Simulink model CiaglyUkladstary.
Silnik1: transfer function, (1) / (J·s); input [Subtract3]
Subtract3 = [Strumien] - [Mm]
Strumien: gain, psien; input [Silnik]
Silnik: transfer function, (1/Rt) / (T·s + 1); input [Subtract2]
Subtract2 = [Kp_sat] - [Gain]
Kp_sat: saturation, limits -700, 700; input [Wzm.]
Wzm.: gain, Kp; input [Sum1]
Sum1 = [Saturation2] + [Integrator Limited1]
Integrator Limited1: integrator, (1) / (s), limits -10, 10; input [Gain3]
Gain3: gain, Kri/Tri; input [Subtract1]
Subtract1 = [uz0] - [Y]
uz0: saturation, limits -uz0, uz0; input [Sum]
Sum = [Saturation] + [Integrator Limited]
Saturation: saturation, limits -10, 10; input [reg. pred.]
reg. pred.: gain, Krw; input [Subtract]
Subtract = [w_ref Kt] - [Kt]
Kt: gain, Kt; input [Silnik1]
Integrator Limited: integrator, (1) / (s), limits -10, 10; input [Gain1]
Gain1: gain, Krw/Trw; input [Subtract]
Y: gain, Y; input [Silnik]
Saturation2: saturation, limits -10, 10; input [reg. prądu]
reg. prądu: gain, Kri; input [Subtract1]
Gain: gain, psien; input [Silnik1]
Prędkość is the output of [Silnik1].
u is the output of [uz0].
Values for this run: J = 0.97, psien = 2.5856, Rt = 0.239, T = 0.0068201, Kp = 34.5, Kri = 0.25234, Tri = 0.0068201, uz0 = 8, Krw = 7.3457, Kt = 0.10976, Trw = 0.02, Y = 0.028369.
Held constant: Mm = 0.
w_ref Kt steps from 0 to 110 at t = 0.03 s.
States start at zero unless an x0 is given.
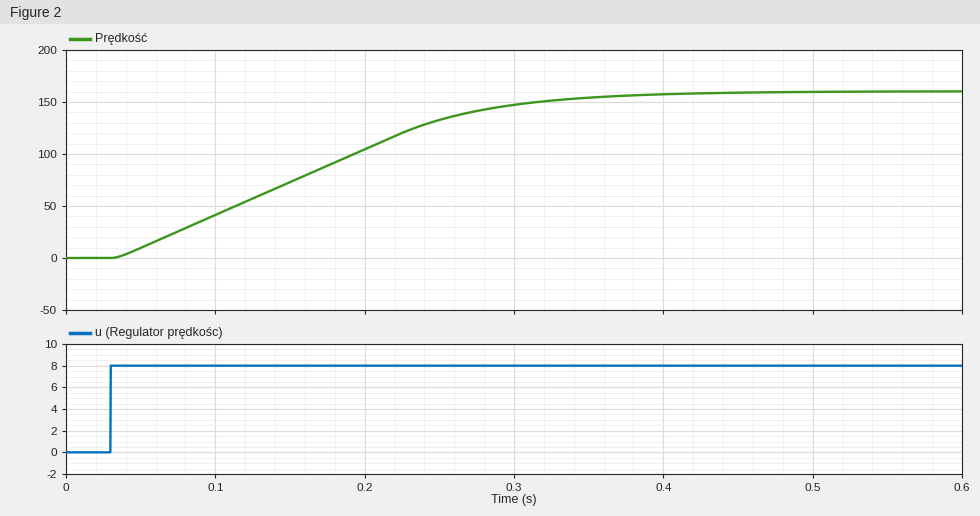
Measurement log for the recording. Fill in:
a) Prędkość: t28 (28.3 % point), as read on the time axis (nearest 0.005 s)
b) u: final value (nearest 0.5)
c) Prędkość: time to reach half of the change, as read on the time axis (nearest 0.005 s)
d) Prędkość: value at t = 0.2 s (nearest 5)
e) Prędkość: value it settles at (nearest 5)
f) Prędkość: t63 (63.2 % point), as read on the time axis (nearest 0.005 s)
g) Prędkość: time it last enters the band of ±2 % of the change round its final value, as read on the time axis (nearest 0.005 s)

0.105 s
8.0
0.160 s
105
160
0.195 s
0.395 s
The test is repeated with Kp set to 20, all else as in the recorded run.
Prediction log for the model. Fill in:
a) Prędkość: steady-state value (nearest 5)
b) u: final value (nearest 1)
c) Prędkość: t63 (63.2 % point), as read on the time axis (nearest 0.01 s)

95
8
0.14 s
